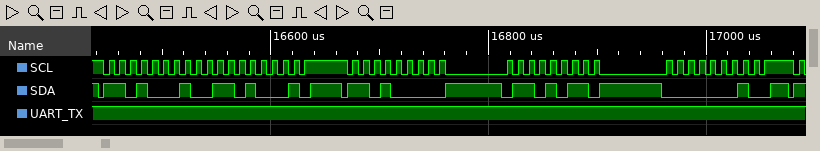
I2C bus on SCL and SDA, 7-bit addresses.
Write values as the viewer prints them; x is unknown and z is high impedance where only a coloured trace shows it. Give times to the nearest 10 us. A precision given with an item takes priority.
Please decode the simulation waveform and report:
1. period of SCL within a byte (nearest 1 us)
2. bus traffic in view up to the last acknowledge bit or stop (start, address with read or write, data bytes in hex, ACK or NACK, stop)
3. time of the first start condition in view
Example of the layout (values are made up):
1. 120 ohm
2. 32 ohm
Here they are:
1. 10 us
2. start, address 68 read ACK, 68 NACK, stop, start, address 68 write ACK, 6B ACK, 01 ACK, stop
3. 16440 us
